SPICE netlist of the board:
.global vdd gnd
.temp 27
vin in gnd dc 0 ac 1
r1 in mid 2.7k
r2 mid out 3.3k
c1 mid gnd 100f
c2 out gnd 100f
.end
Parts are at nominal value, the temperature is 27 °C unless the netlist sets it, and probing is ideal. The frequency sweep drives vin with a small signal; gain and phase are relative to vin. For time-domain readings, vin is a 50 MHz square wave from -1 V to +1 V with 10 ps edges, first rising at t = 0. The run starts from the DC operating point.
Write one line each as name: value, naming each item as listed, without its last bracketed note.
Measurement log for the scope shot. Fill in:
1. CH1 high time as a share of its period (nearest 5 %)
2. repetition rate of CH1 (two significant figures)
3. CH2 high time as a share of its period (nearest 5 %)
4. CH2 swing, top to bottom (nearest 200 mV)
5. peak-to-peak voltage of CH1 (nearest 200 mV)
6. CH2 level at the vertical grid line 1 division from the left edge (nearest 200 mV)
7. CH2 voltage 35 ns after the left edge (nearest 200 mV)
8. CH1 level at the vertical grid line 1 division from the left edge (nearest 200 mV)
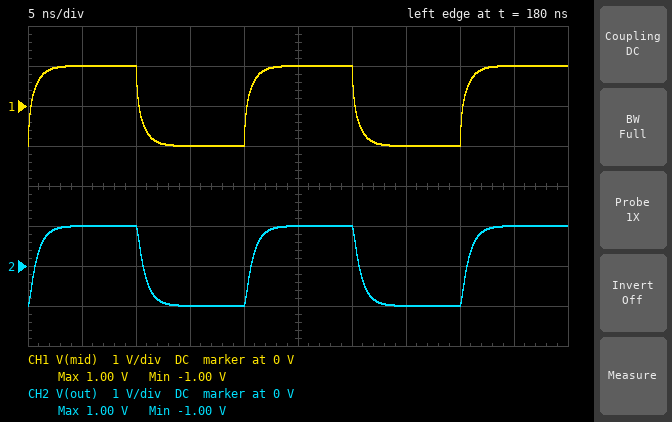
CH1 high time as a share of its period: 50 %
repetition rate of CH1: 50 MHz
CH2 high time as a share of its period: 50 %
CH2 swing, top to bottom: 2.0 V
peak-to-peak voltage of CH1: 2.0 V
CH2 level at the vertical grid line 1 division from the left edge: 1.0 V
CH2 voltage 35 ns after the left edge: -1.0 V
CH1 level at the vertical grid line 1 division from the left edge: 1.0 V
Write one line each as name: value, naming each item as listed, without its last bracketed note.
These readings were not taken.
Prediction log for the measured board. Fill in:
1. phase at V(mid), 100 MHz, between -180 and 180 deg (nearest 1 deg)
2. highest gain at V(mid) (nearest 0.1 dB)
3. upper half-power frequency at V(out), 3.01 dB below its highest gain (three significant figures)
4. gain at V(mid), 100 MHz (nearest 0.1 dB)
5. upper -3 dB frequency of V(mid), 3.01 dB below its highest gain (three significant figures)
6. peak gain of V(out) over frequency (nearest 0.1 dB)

phase at V(mid), 100 MHz, between -180 and 180 deg: -18 deg
highest gain at V(mid): 0 dB
upper half-power frequency at V(out), 3.01 dB below its highest gain: 207 MHz
gain at V(mid), 100 MHz: -0.7 dB
upper -3 dB frequency of V(mid), 3.01 dB below its highest gain: 258 MHz
peak gain of V(out) over frequency: 0 dB
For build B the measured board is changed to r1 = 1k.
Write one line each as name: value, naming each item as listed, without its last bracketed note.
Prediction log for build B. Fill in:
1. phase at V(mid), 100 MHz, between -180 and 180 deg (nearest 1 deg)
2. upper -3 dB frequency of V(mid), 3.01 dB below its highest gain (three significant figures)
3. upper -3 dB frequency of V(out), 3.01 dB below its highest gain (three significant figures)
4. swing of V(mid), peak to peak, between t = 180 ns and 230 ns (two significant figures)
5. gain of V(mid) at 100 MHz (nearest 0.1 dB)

phase at V(mid), 100 MHz, between -180 and 180 deg: -7 deg
upper -3 dB frequency of V(mid), 3.01 dB below its highest gain: 896 MHz
upper -3 dB frequency of V(out), 3.01 dB below its highest gain: 339 MHz
swing of V(mid), peak to peak, between t = 180 ns and 230 ns: 2.0 V
gain of V(mid) at 100 MHz: -0.2 dB
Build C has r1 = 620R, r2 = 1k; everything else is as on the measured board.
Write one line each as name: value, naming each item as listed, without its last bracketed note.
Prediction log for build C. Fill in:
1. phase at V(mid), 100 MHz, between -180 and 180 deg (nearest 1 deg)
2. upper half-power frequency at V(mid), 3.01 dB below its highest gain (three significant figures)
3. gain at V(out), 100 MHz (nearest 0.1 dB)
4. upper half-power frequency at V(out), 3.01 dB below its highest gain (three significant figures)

phase at V(mid), 100 MHz, between -180 and 180 deg: -4 deg
upper half-power frequency at V(mid), 3.01 dB below its highest gain: 1.13 GHz
gain at V(out), 100 MHz: -0.1 dB
upper half-power frequency at V(out), 3.01 dB below its highest gain: 808 MHz
